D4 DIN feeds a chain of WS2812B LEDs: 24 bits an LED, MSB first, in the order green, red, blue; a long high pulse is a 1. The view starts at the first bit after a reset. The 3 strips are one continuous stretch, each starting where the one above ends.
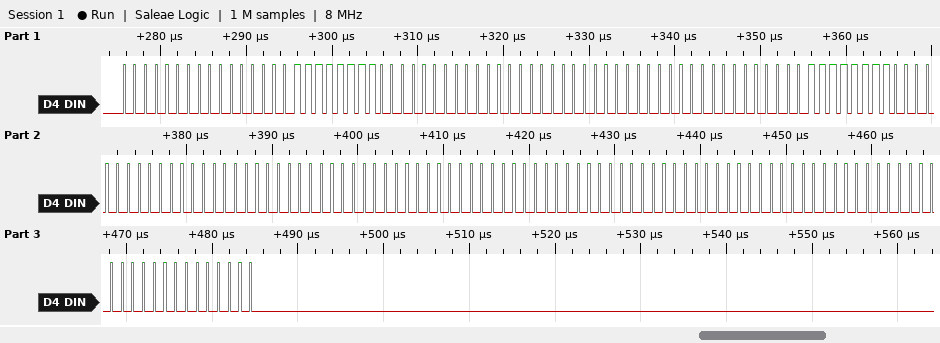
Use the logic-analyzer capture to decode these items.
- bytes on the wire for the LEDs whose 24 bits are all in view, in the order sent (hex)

00 00 FF 00 00 00 00 00 FF 00 00 00 00 00 00 00 00 00 00 00 00
